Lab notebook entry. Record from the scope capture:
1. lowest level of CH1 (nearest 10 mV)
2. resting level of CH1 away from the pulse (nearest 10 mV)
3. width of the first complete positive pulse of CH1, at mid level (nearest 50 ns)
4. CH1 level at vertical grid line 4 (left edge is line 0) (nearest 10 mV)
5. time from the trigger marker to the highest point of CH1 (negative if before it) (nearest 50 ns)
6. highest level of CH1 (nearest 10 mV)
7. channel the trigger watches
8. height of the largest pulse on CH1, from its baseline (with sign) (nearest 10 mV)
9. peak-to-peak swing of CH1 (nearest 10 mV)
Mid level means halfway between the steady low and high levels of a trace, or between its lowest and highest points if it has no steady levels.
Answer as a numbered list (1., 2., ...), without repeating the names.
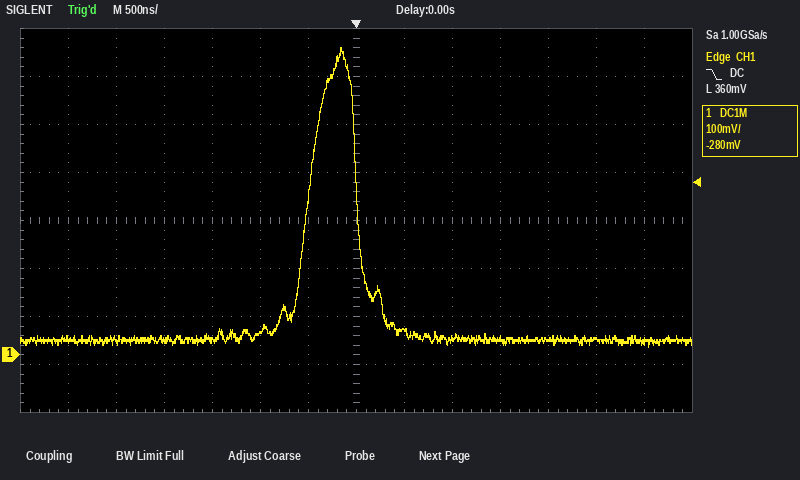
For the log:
1. 20 mV
2. 30 mV
3. 500 ns
4. 30 mV
5. -150 ns
6. 640 mV
7. CH1
8. +610 mV
9. 620 mV
